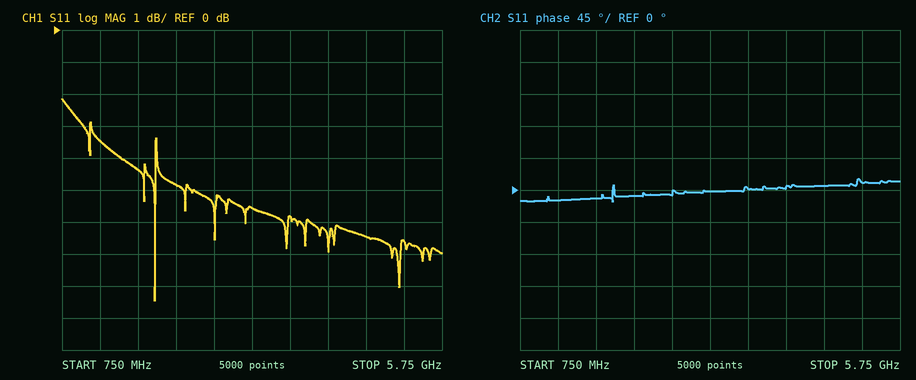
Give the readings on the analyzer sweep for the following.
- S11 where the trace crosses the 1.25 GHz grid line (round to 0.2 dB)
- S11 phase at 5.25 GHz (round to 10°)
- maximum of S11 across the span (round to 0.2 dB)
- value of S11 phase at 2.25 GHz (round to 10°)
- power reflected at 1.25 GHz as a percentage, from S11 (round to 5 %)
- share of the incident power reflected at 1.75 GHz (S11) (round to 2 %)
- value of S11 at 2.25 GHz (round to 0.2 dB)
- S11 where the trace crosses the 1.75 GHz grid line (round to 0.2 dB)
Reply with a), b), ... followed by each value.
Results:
a) -3.4 dB
b) 10°
c) -2.2 dB
d) -10°
e) 45 %
f) 36 %
g) -4.8 dB
h) -4.4 dB
